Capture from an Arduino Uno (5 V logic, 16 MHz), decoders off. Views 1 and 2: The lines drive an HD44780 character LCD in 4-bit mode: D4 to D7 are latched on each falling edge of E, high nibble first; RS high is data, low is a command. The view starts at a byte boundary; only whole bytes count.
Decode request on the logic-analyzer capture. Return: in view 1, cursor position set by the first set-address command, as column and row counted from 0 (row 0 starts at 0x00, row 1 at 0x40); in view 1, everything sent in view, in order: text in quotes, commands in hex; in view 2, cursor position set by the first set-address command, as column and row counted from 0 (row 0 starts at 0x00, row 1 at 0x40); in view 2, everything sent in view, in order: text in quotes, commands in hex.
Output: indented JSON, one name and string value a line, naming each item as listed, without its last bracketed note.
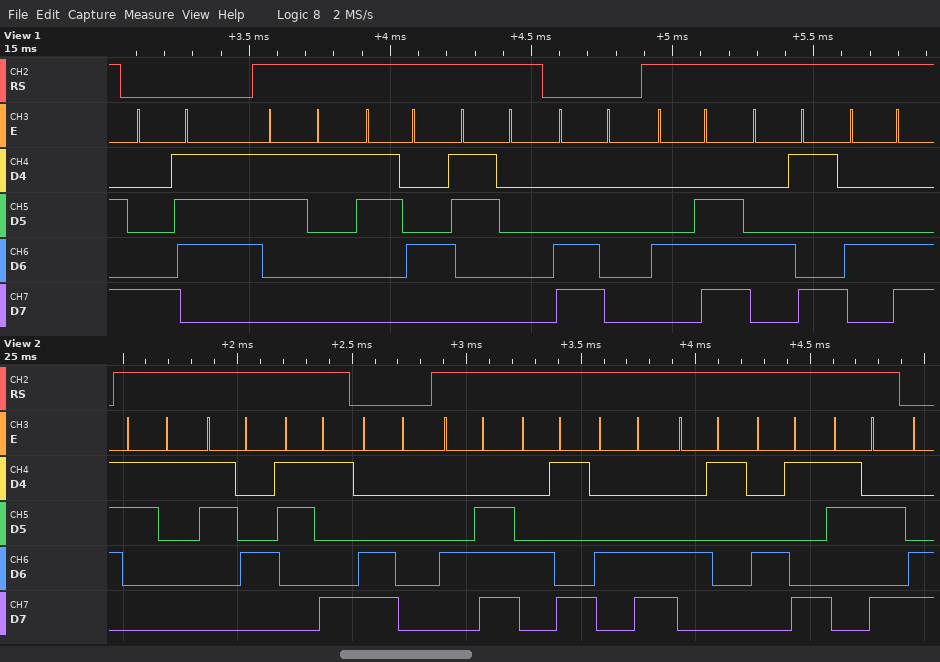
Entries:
{
  "in view 1, cursor position set by the first set-address command, as column and row counted from 0": "column 7, row 0",
  "in view 1, everything sent in view, in order: text in quotes, commands in hex": "0x87 \"140\" 0xC0 \"NIL\"",
  "in view 2, cursor position set by the first set-address command, as column and row counted from 0": "column 0, row 1",
  "in view 2, everything sent in view, in order: text in quotes, commands in hex": "\"149\" 0xC0 \"NILAI:\""
}
